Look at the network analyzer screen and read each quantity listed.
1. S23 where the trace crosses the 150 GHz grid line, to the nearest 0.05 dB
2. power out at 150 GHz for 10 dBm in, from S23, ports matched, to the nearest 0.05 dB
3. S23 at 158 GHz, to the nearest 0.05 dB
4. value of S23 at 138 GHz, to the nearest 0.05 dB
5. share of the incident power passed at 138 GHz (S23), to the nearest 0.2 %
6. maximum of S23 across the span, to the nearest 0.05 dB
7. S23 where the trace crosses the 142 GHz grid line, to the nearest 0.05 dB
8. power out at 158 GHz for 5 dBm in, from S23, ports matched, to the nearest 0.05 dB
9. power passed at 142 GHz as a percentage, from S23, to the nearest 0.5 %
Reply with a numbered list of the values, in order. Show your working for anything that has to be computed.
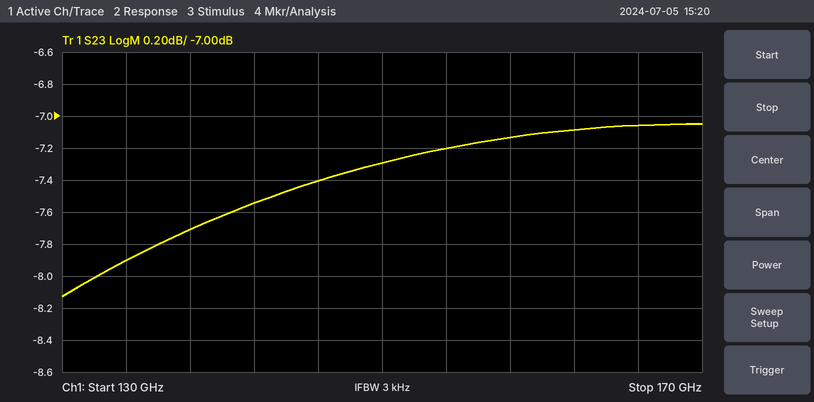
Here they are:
1. -7.30 dB
2. 10 dBm + (-7.30 dB) = 2.70 dBm
3. -7.15 dB
4. -7.70 dB
5. 10^(-7.7/10) ≈ 17.0 %
6. -7.05 dB
7. -7.55 dB
8. 5 dBm + (-7.15 dB) = -2.15 dBm
9. 10^(-7.55/10) ≈ 17.6 %, so 17.5 % to the nearest 0.5 %
